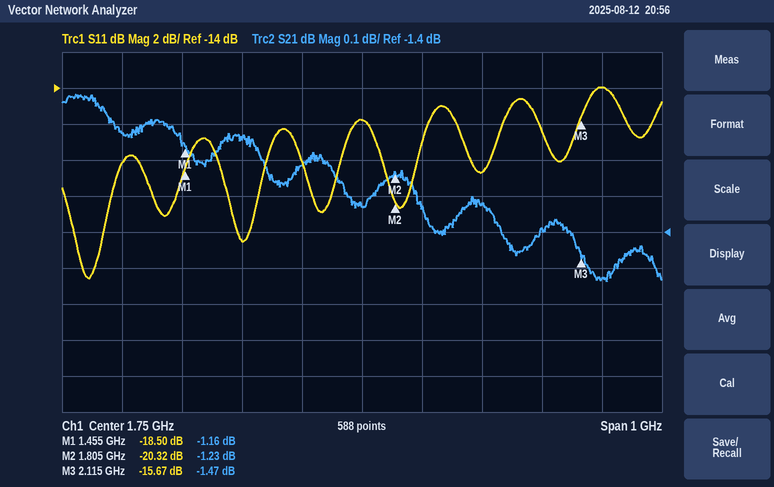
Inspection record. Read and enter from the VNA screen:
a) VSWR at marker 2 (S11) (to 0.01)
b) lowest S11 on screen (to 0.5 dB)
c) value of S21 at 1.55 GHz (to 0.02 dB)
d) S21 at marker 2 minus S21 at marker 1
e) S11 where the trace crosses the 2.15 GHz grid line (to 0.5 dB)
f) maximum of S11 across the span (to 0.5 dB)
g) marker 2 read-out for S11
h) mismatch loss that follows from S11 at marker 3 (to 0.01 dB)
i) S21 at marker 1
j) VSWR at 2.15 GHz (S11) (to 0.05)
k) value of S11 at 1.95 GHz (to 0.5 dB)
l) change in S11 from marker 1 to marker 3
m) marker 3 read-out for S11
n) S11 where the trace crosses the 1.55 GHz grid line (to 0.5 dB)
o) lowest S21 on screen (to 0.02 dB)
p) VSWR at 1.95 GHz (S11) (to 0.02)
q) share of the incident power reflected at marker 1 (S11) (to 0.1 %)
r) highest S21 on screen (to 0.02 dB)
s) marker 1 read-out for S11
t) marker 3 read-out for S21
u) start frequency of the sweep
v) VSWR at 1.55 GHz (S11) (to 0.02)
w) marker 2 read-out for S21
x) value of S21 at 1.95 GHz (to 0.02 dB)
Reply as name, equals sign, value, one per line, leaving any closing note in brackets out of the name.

VSWR at marker 2 (S11) = 1.21
lowest S11 on screen = -24.5 dB
value of S21 at 1.55 GHz = -1.14 dB
S21 at marker 2 minus S21 at marker 1 = -0.07 dB
S11 where the trace crosses the 2.15 GHz grid line = -14.0 dB
maximum of S11 across the span = -14.0 dB
marker 2 read-out for S11 = -20.32 dB
mismatch loss that follows from S11 at marker 3 = 0.12 dB
S21 at marker 1 = -1.16 dB
VSWR at 2.15 GHz (S11) = 1.50
value of S11 at 1.95 GHz = -18.5 dB
change in S11 from marker 1 to marker 3 = 2.83 dB
marker 3 read-out for S11 = -15.67 dB
S11 where the trace crosses the 1.55 GHz grid line = -22.5 dB
lowest S21 on screen = -1.54 dB
VSWR at 1.95 GHz (S11) = 1.26
share of the incident power reflected at marker 1 (S11) = 1.4 %
highest S21 on screen = -1.02 dB
marker 1 read-out for S11 = -18.50 dB
marker 3 read-out for S21 = -1.47 dB
start frequency of the sweep = 1.25 GHz
VSWR at 1.55 GHz (S11) = 1.16
marker 2 read-out for S21 = -1.23 dB
value of S21 at 1.95 GHz = -1.32 dB
